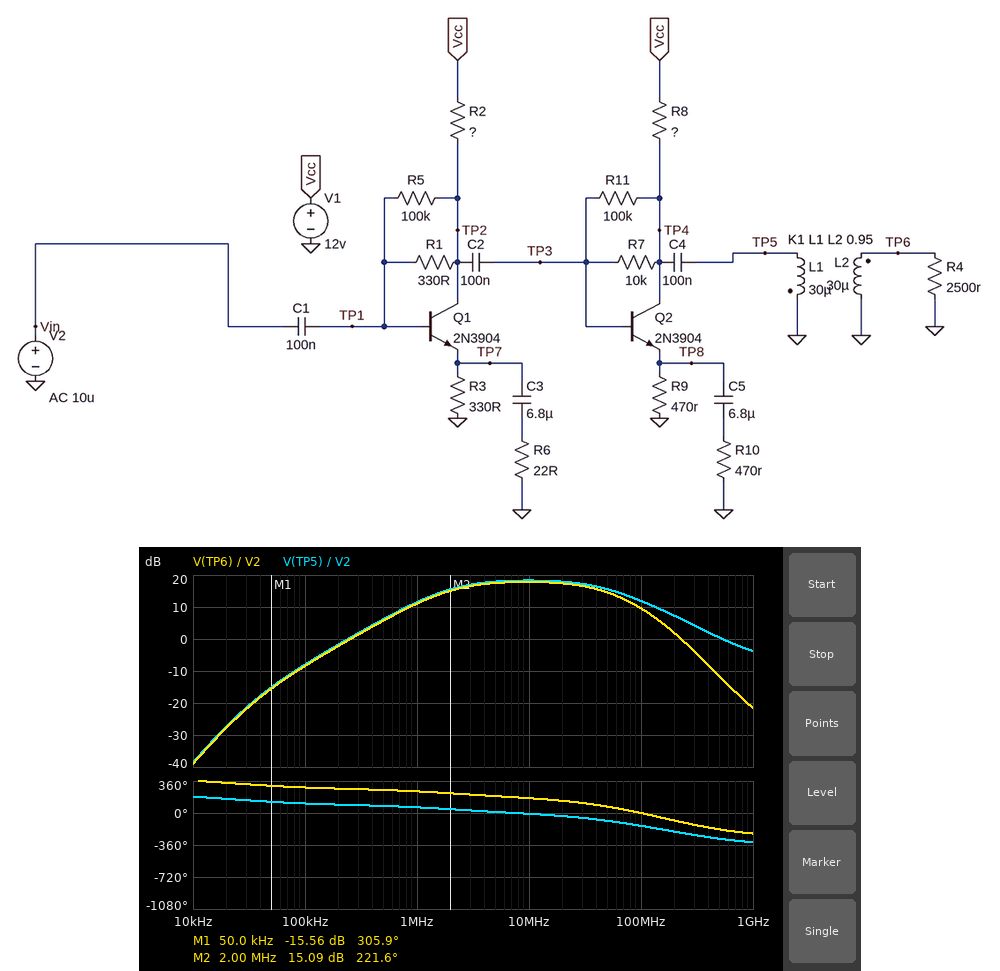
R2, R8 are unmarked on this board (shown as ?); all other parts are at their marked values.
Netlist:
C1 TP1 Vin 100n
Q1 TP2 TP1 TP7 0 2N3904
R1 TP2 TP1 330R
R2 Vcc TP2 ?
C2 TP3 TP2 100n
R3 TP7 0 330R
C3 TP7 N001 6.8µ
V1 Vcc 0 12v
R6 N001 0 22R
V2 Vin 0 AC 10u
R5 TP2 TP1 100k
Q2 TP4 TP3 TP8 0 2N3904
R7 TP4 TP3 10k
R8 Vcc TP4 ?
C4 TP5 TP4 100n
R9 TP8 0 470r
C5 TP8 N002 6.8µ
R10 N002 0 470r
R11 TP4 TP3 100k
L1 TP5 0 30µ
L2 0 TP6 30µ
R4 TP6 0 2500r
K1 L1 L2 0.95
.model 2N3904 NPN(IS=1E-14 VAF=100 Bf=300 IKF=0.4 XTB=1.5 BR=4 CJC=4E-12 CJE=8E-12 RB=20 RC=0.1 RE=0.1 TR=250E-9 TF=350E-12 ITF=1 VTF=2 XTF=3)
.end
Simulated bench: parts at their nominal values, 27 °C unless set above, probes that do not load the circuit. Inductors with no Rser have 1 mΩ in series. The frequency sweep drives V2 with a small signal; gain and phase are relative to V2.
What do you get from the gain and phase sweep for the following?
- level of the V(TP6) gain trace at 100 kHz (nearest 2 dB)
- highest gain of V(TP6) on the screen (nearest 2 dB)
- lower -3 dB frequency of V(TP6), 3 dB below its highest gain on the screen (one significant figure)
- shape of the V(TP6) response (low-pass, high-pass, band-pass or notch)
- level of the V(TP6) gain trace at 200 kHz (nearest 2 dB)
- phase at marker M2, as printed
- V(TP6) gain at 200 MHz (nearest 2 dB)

-8 dB
18 dB
2 MHz
band-pass
-2 dB
221.6 deg
2 dB
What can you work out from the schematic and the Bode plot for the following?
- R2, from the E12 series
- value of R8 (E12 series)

220 Ω
470 Ω
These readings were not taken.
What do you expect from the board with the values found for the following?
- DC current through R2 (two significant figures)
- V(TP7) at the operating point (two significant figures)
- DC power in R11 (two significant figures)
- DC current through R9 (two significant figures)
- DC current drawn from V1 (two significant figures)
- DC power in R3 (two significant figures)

20 mA
6.7 V
1.3 µW
12 mA
32 mA
140 mW
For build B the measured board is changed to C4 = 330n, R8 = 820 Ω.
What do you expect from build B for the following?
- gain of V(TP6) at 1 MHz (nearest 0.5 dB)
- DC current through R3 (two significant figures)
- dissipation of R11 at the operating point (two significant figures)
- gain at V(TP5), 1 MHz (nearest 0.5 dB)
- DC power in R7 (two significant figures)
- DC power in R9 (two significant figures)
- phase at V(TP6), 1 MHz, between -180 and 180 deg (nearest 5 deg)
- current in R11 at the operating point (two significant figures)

11.5 dB
20 mA
690 nW
12.0 dB
6.9 µW
34 mW
-110 deg
2.6 µA
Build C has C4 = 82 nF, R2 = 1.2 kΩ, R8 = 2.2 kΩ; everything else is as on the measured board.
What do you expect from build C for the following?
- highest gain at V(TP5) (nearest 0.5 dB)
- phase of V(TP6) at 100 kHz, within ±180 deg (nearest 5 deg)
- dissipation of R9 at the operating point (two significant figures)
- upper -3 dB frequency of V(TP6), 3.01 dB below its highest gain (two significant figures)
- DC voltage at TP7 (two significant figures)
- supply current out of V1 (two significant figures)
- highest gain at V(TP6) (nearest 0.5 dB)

30.5 dB
-65 deg
8.2 mW
22 MHz
2.4 V
12 mA
30.0 dB
